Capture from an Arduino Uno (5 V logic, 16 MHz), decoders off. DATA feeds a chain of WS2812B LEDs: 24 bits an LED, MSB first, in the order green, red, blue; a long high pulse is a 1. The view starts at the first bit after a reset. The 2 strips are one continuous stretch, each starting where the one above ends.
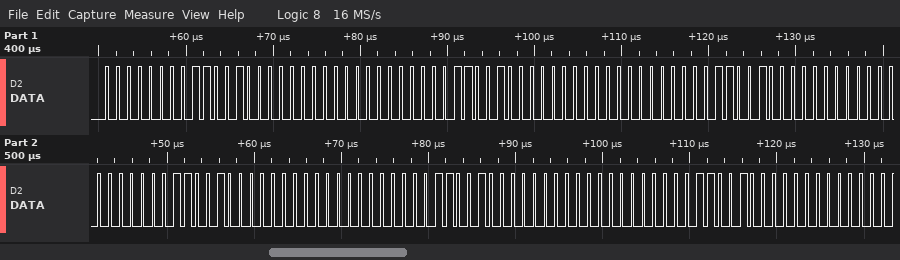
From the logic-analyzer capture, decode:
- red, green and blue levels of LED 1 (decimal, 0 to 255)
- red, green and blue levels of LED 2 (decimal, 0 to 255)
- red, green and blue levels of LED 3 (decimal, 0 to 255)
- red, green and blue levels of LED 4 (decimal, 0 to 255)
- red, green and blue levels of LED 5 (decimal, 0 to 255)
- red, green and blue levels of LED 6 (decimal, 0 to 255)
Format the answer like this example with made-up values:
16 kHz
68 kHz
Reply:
200, 0, 0
200, 0, 0
200, 0, 0
200, 0, 0
200, 0, 0
200, 0, 0
